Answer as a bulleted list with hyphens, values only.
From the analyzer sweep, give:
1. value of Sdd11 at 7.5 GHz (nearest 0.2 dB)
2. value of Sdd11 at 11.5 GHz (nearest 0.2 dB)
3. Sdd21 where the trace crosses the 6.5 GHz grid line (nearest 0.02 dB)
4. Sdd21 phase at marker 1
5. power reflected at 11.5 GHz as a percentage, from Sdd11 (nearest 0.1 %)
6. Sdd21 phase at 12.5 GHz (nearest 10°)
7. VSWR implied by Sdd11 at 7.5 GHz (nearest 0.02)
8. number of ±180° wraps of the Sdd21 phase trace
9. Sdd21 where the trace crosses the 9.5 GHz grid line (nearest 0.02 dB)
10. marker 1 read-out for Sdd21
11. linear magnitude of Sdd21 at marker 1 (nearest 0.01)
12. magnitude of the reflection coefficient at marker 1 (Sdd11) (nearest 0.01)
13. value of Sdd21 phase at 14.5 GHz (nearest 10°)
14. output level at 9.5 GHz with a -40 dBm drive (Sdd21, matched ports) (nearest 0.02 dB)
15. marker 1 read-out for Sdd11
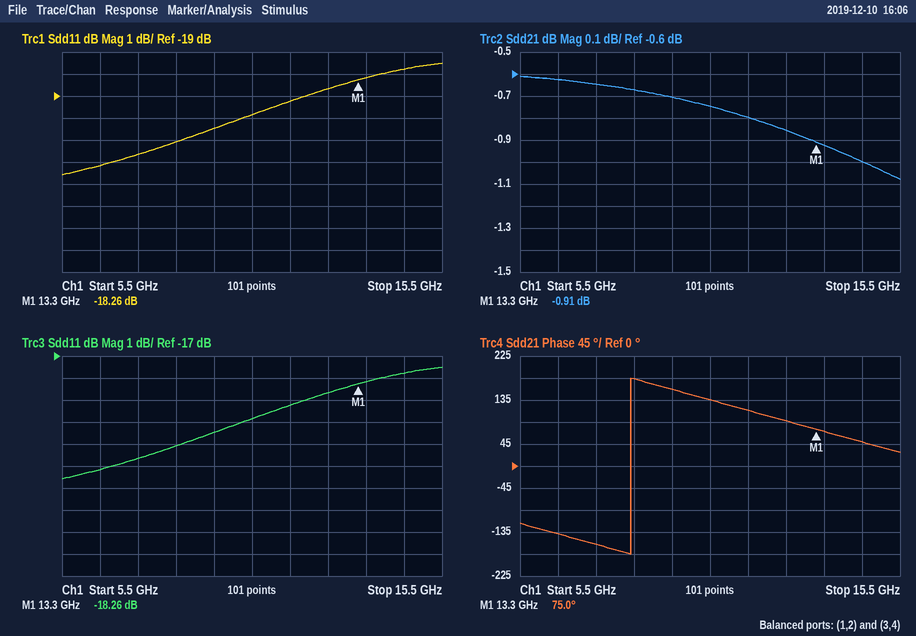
- -21.6 dB
- -19.2 dB
- -0.62 dB
- 75.0°
- 1.2 %
- 90°
- 1.18
- 1
- -0.70 dB
- -0.91 dB
- 0.90
- 0.12
- 50°
- -40.70 dBm
- -18.26 dB
